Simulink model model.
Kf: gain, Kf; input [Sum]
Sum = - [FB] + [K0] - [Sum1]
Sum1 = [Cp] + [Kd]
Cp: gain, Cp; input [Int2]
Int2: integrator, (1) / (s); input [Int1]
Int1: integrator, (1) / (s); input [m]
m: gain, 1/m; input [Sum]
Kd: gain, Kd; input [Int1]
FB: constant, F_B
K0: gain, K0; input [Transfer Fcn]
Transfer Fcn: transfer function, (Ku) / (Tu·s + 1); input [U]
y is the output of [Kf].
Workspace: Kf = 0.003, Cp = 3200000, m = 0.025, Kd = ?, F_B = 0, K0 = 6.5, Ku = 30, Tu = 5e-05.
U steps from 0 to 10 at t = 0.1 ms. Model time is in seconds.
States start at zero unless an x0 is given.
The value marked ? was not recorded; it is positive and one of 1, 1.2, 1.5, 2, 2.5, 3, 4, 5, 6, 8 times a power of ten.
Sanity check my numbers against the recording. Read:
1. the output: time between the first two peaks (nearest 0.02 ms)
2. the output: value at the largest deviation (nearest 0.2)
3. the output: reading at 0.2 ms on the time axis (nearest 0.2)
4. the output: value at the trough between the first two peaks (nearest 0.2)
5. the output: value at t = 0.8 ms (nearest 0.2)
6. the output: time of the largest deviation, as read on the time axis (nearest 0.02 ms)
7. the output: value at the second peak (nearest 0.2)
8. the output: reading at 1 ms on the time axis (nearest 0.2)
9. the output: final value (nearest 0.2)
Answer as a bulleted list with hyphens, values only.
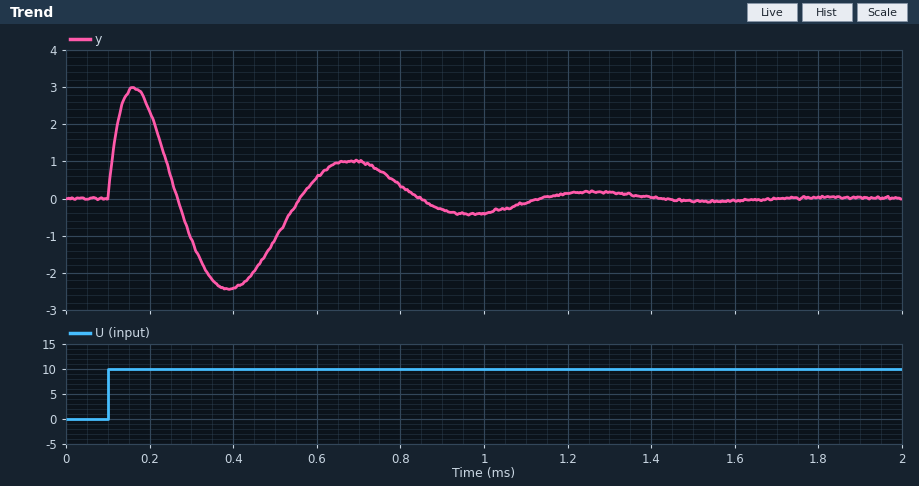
- 0.52 ms
- 3.0
- 2.4
- -2.4
- 0.4
- 0.16 ms
- 1.0
- -0.4
- 0.0
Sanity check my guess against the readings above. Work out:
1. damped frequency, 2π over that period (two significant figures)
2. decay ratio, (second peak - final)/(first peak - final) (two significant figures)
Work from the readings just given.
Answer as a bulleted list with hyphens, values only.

- 12 rad/ms
- 0.33
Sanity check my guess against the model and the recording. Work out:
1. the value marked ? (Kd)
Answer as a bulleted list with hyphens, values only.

- 150
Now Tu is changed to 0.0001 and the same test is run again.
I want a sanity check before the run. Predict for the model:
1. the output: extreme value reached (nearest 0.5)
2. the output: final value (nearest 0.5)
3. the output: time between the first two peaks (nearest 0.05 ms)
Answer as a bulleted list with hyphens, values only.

- 2.0
- 0.0
- 0.55 ms
